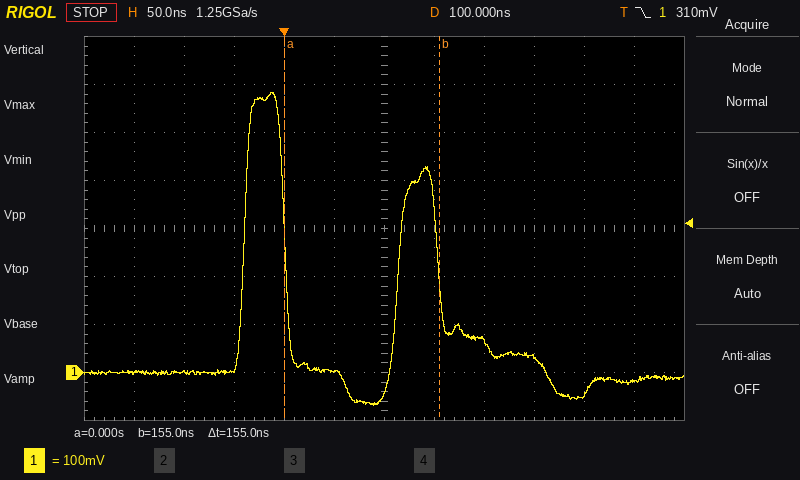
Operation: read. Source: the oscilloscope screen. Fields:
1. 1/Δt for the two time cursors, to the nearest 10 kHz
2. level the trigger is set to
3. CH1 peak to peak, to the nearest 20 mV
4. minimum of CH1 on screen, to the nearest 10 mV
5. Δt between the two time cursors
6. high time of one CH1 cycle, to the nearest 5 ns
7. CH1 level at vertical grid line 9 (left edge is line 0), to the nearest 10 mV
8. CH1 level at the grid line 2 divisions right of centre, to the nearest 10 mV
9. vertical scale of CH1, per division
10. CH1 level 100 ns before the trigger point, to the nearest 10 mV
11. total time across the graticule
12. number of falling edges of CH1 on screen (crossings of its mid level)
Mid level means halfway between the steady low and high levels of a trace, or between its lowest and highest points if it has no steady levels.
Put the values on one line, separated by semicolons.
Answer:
6.45 MHz; 310 mV; 660 mV; -70 mV; 155 ns; 40 ns; 30 mV; 70 mV; 100 mV; 0 mV; 600 ns; 2
